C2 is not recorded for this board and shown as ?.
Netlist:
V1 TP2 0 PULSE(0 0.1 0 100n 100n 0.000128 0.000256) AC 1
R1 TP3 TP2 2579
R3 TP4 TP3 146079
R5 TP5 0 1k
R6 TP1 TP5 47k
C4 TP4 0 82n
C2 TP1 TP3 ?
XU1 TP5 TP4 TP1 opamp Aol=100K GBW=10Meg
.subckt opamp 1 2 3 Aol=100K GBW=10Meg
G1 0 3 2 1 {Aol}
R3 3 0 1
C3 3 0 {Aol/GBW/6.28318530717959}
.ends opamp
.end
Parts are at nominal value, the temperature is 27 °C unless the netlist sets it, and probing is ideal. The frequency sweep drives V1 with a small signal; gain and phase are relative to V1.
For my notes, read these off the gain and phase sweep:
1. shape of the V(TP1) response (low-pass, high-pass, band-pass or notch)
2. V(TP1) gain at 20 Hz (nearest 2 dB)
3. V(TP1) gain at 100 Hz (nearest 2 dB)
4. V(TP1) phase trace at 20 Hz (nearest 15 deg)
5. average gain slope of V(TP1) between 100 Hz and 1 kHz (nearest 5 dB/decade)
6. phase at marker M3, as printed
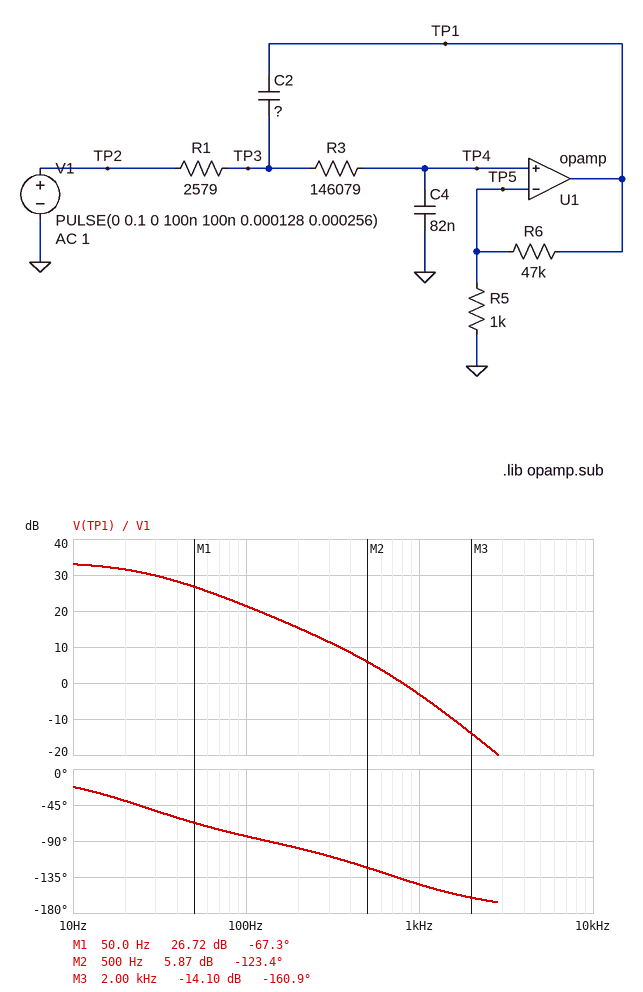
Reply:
low-pass
32 dB
22 dB
-45 deg
-25 dB/decade
-160.9 deg
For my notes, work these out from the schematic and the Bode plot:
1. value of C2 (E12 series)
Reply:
47 nF
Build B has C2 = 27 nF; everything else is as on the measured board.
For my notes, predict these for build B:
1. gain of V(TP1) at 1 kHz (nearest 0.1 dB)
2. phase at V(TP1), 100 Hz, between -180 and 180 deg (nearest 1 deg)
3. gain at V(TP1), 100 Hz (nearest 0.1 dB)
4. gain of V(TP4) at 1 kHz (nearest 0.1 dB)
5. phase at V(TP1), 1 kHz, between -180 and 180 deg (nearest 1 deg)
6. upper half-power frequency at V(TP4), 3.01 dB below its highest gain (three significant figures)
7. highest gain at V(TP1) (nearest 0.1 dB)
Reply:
-2.6 dB
-83 deg
18.6 dB
-36.2 dB
-120 deg
18.0 Hz
33.6 dB
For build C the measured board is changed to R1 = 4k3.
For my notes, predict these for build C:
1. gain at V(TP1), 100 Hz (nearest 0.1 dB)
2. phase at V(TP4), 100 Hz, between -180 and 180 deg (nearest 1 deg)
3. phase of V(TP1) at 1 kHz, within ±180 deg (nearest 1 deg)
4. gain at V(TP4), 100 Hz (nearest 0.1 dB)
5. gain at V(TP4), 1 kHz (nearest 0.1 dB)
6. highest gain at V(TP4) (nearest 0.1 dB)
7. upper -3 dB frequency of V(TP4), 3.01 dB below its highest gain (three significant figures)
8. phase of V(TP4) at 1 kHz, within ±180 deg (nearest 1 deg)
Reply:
28.6 dB
-89 deg
-170 deg
-5.0 dB
-39.7 dB
0 dB
75.0 Hz
-169 deg
